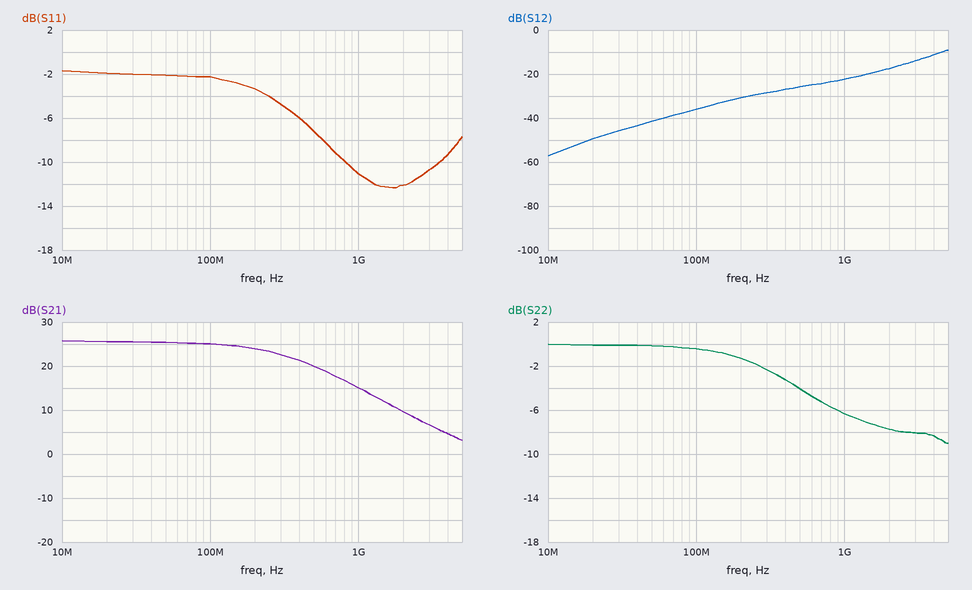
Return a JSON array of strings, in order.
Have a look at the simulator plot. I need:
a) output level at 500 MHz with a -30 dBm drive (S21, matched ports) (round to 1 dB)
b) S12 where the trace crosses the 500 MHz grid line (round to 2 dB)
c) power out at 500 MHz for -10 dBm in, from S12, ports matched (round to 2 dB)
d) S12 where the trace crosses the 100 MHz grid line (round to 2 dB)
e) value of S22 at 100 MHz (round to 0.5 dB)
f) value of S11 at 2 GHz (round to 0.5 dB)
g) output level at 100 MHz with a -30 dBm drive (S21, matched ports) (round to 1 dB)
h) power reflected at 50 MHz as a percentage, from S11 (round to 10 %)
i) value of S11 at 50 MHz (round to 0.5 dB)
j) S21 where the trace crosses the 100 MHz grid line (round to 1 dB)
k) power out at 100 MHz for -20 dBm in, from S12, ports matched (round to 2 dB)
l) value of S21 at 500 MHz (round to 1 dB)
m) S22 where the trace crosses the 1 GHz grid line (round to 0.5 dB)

["-10 dBm", "-26 dB", "-36 dBm", "-36 dB", "-0.5 dB", "-12.0 dB", "-5 dBm", "60 %", "-2.0 dB", "25 dB", "-56 dBm", "20 dB", "-6.5 dB"]
